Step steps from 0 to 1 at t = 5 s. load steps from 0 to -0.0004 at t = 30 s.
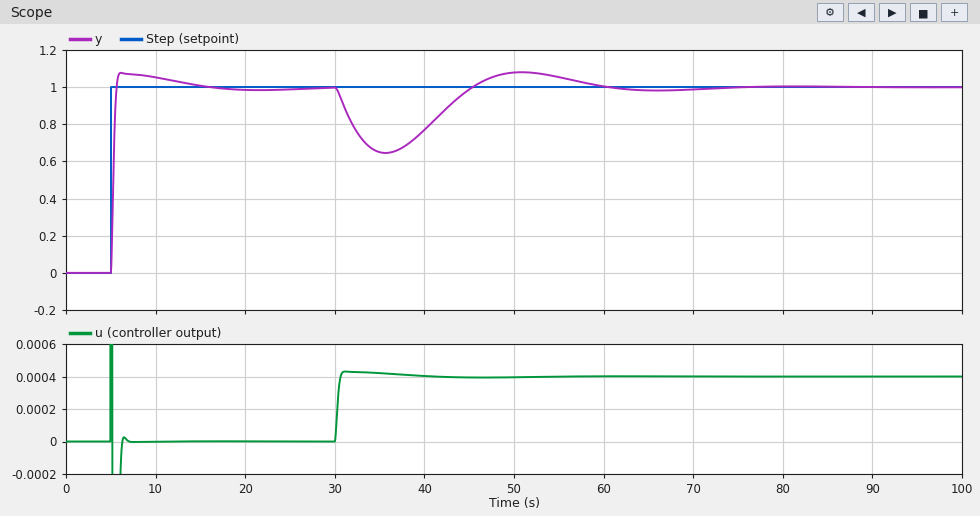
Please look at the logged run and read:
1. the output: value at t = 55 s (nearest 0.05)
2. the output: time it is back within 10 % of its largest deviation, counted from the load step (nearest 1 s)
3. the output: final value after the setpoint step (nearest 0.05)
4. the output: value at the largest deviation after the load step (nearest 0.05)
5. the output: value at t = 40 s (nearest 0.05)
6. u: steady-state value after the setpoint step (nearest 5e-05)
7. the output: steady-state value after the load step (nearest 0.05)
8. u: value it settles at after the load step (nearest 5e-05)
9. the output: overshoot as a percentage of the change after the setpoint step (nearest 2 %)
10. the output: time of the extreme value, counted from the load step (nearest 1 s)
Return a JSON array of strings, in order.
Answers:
["1.05", "27 s", "1.00", "0.65", "0.75", "0.00000", "1.00", "0.00040", "8 %", "6 s"]
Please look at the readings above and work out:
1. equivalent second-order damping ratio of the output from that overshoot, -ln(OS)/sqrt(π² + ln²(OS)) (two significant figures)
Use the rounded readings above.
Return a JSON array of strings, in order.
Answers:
["0.63"]
